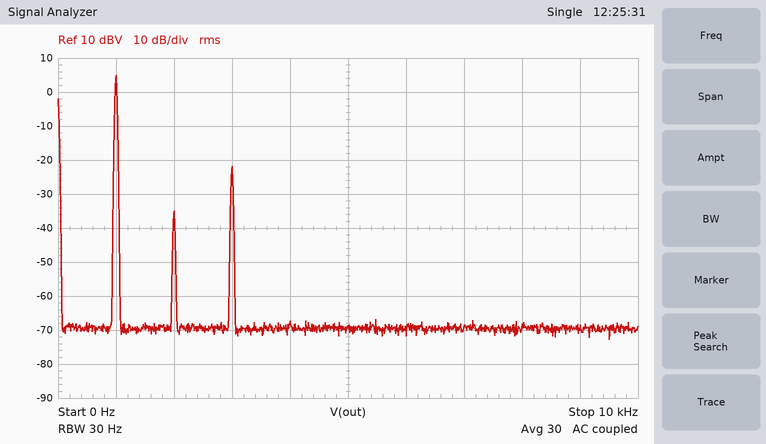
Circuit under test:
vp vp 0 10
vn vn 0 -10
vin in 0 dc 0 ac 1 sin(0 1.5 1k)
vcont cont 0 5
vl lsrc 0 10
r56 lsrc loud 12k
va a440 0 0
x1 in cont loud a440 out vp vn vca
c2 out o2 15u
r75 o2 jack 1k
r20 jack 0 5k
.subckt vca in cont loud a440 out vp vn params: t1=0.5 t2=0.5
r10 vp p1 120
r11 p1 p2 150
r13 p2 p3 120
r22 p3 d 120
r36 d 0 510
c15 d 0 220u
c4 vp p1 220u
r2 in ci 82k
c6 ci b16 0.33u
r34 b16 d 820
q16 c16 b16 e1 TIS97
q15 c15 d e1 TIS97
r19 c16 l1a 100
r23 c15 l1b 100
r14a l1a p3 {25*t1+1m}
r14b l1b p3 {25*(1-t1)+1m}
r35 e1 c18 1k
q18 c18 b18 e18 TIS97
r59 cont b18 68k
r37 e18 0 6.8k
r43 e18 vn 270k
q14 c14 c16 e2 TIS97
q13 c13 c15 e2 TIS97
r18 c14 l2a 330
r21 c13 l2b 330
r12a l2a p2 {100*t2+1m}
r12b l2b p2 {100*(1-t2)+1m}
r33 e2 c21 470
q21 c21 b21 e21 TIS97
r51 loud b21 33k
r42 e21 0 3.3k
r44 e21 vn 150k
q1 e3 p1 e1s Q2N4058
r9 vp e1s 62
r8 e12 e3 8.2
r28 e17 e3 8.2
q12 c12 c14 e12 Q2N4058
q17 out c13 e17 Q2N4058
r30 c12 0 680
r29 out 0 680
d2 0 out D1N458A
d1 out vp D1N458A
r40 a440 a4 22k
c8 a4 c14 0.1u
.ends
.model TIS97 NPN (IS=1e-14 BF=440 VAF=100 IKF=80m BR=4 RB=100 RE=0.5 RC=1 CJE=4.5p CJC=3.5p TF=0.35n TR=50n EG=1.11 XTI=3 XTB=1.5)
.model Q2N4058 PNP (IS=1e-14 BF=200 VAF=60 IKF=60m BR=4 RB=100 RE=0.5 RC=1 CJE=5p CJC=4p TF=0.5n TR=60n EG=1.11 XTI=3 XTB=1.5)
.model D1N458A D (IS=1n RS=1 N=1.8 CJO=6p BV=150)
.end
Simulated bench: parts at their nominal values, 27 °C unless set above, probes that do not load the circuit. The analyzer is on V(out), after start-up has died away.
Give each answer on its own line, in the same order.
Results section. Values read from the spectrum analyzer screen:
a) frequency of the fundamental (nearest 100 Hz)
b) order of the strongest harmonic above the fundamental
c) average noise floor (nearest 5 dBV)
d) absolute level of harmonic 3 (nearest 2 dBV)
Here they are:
1.0 kHz
3
-70 dBV
-22 dBV
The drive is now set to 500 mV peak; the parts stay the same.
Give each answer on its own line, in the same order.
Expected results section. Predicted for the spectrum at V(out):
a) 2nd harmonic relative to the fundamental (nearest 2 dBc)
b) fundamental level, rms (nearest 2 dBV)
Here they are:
-50 dBc
-4 dBV
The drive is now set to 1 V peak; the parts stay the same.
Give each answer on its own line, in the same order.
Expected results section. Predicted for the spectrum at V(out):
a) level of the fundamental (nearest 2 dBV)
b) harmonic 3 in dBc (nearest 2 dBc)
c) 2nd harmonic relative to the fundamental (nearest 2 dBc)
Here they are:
2 dBV
-34 dBc
-44 dBc
